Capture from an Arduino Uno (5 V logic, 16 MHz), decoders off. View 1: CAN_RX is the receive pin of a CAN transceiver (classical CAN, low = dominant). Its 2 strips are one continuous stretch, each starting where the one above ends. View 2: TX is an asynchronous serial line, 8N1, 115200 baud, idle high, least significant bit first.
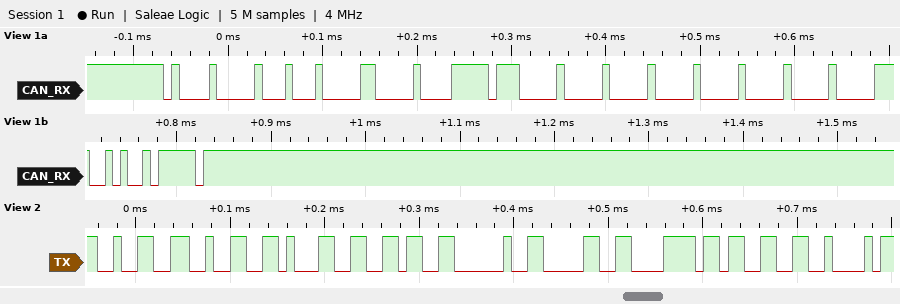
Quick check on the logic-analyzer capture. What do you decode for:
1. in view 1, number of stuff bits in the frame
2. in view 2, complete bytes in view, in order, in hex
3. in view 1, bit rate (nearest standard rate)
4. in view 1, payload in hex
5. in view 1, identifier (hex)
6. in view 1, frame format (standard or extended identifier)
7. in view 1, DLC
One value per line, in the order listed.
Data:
12
0x32 0x32 0x31 0x36 0x20 0x30 0x78 0x33 0x42
125 kbit/s
82 00 FF 00 00 00 00 00
0x420
standard
8
